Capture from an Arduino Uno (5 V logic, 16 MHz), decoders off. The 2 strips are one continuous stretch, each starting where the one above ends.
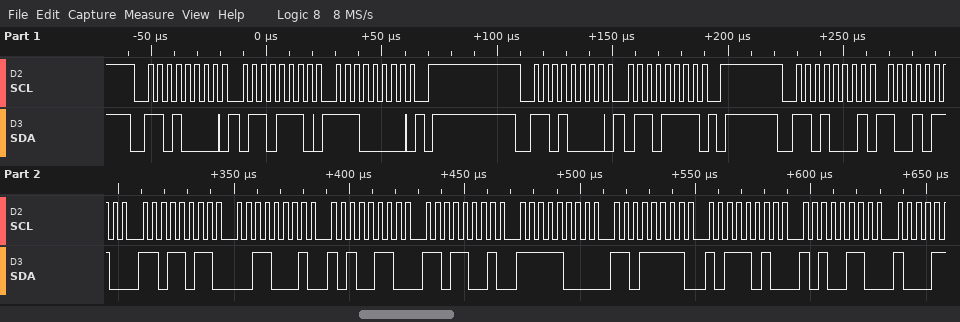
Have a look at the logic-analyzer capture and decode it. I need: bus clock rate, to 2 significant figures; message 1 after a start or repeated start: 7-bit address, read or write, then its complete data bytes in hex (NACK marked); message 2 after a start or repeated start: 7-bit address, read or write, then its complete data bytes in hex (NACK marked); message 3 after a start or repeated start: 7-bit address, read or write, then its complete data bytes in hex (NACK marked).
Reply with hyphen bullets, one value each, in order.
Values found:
- 250 kHz
- 0x68 write: 6E E0
- 0x68 write: 6F
- 0x68 read: 96 DB 31 A6 D9 F8 DF BA A6
